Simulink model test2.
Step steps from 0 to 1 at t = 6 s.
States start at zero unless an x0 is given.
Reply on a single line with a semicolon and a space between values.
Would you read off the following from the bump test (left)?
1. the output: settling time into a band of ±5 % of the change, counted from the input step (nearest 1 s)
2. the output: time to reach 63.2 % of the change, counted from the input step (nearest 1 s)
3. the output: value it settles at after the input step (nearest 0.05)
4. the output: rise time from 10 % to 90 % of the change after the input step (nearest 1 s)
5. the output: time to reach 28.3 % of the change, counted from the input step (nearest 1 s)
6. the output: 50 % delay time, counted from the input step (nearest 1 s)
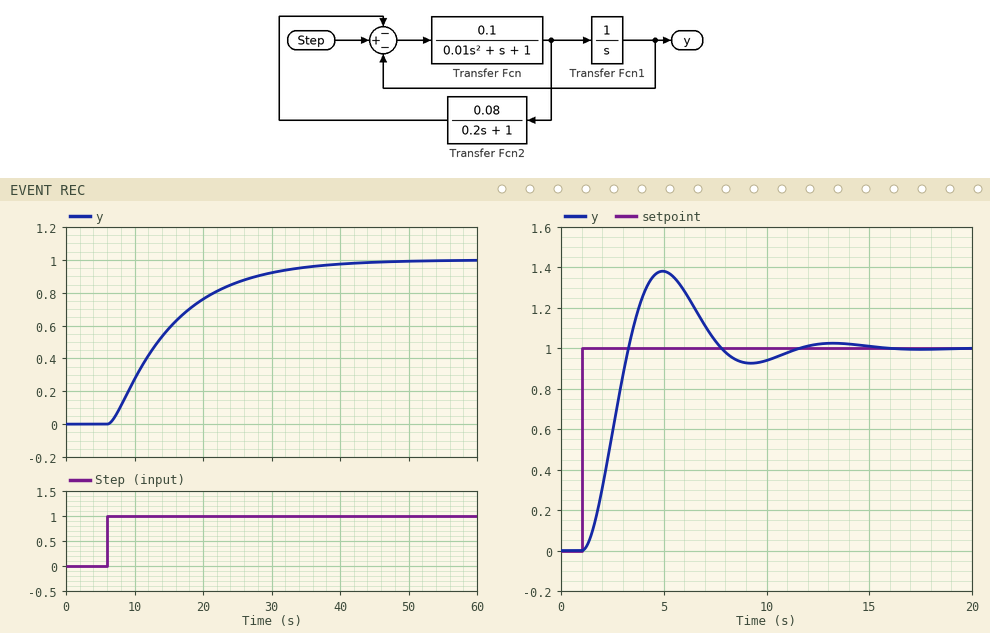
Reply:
28 s; 10 s; 1.00; 20 s; 4 s; 7 s
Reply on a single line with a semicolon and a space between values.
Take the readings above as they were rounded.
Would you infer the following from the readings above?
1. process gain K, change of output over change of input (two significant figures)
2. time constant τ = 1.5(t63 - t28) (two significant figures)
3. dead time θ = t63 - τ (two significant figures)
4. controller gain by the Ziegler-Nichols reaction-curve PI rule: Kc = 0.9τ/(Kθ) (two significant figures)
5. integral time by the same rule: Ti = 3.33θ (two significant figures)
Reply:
1.0; 9.0 s; 1.0 s; 8.1; 3.3 s
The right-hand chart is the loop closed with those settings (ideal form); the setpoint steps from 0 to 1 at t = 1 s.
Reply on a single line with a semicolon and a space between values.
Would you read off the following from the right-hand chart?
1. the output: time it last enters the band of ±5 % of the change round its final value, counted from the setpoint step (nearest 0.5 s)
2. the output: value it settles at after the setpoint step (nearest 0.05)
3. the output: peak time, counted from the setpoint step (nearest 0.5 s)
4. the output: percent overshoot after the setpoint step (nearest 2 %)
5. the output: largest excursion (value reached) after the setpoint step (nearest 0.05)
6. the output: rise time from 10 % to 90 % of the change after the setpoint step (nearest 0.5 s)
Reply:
9.5 s; 1.00; 4.0 s; 38 %; 1.40; 1.5 s
